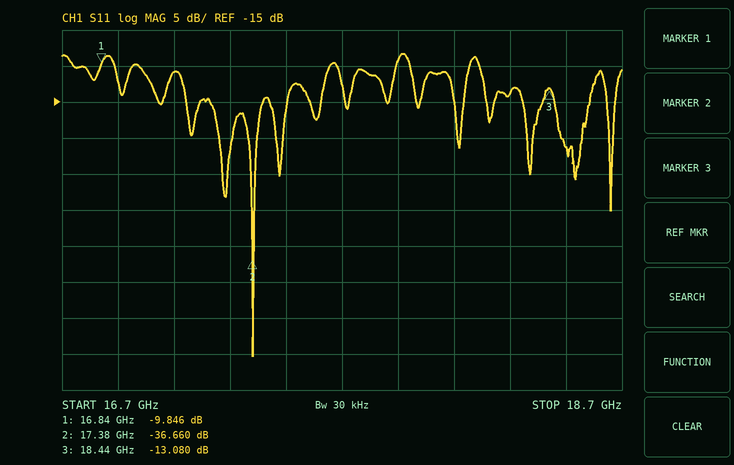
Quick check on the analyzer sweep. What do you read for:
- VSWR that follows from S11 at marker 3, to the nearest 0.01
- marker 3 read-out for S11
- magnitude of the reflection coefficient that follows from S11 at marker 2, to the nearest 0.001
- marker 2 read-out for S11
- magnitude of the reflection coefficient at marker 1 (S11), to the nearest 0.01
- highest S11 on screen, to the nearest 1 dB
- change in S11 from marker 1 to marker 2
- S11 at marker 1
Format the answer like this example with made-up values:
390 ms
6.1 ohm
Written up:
1.57
-13.080 dB
0.015
-36.660 dB
0.32
-8 dB
-26.814 dB
-9.846 dB
